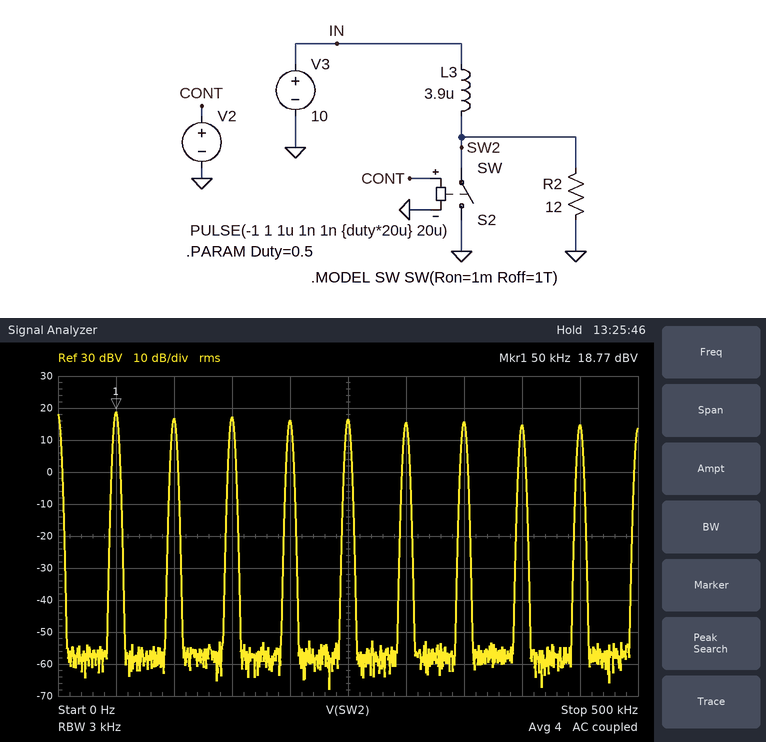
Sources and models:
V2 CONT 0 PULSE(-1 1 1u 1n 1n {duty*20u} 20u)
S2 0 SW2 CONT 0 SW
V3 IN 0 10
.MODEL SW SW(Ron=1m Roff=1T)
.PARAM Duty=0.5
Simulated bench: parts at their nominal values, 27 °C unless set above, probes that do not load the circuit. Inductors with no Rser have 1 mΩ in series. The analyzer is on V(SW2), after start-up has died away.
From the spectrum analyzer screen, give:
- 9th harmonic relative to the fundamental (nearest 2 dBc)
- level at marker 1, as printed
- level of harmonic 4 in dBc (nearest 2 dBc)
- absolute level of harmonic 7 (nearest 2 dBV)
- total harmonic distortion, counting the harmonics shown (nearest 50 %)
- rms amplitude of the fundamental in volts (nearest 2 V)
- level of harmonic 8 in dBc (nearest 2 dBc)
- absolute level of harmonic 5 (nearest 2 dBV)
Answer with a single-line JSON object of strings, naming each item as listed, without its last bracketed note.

{"9th harmonic relative to the fundamental": "-4 dBc", "level at marker 1, as printed": "18.77 dBV", "level of harmonic 4 in dBc": "-2 dBc", "absolute level of harmonic 7": "16 dBV", "total harmonic distortion, counting the harmonics shown": "200 %", "rms amplitude of the fundamental in volts": "8 V", "level of harmonic 8 in dBc": "-4 dBc", "absolute level of harmonic 5": "16 dBV"}
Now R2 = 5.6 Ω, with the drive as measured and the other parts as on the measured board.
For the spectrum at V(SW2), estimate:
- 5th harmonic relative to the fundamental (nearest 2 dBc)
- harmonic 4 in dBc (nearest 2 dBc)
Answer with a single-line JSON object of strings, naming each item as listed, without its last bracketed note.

{"5th harmonic relative to the fundamental": "-4 dBc", "harmonic 4 in dBc": "-4 dBc"}
